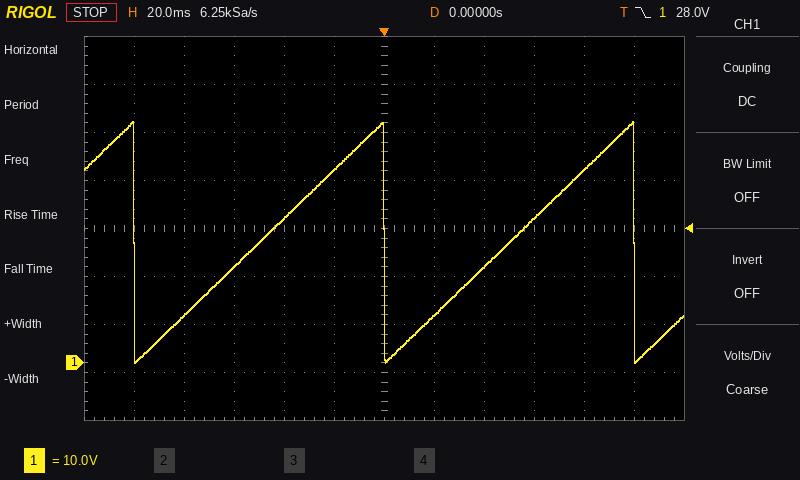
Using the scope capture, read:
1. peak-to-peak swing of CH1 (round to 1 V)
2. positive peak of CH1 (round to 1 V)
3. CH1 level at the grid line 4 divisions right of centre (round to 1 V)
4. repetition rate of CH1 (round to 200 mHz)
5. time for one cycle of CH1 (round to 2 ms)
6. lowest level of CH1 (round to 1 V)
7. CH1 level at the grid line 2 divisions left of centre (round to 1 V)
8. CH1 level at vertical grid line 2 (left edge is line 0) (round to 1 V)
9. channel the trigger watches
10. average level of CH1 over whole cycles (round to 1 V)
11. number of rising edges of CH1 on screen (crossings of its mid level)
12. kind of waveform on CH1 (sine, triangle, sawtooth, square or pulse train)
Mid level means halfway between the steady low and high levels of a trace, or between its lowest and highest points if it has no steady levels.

50 V
50 V
40 V
10.0 Hz
100 ms
0 V
30 V
10 V
CH1
25 V
2
sawtooth
